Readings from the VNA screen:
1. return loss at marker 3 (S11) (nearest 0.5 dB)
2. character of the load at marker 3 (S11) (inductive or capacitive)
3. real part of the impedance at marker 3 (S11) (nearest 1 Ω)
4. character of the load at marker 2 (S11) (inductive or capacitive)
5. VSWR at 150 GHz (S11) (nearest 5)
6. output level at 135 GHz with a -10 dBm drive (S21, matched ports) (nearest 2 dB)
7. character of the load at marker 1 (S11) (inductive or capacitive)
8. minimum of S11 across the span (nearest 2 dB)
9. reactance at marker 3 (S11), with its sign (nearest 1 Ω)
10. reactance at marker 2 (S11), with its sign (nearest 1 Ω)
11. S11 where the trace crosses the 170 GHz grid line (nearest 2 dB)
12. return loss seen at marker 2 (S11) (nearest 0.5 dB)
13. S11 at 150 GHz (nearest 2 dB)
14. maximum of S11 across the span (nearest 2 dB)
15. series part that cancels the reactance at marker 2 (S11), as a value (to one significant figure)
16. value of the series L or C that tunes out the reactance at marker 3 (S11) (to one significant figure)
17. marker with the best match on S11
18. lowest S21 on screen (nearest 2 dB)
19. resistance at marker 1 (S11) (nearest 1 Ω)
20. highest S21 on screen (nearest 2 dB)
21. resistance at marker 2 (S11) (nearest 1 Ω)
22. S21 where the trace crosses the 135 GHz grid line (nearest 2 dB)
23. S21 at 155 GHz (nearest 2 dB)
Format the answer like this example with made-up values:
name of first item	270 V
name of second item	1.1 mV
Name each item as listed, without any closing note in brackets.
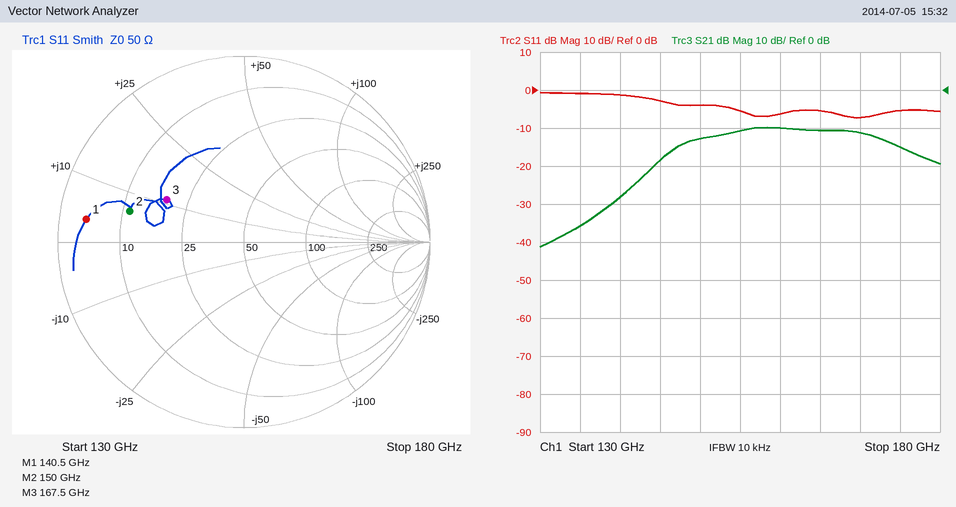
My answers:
return loss at marker 3 (S11)	6.5 dB
character of the load at marker 3 (S11)	inductive
real part of the impedance at marker 3 (S11)	19 Ω
character of the load at marker 2 (S11)	inductive
VSWR at 150 GHz (S11)	5
output level at 135 GHz with a -10 dBm drive (S21, matched ports)	-46 dBm
character of the load at marker 1 (S11)	inductive
minimum of S11 across the span	-8 dB
reactance at marker 3 (S11), with its sign	+11 Ω
reactance at marker 2 (S11), with its sign	+6 Ω
S11 where the trace crosses the 170 GHz grid line	-8 dB
return loss seen at marker 2 (S11)	4.0 dB
S11 at 150 GHz	-4 dB
maximum of S11 across the span	0 dB
series part that cancels the reactance at marker 2 (S11), as a value	200 fF
value of the series L or C that tunes out the reactance at marker 3 (S11)	90 fF
marker with the best match on S11	marker 3
lowest S21 on screen	-42 dB
resistance at marker 1 (S11)	4 Ω
highest S21 on screen	-10 dB
resistance at marker 2 (S11)	11 Ω
S21 where the trace crosses the 135 GHz grid line	-36 dB
S21 at 155 GHz	-10 dB
